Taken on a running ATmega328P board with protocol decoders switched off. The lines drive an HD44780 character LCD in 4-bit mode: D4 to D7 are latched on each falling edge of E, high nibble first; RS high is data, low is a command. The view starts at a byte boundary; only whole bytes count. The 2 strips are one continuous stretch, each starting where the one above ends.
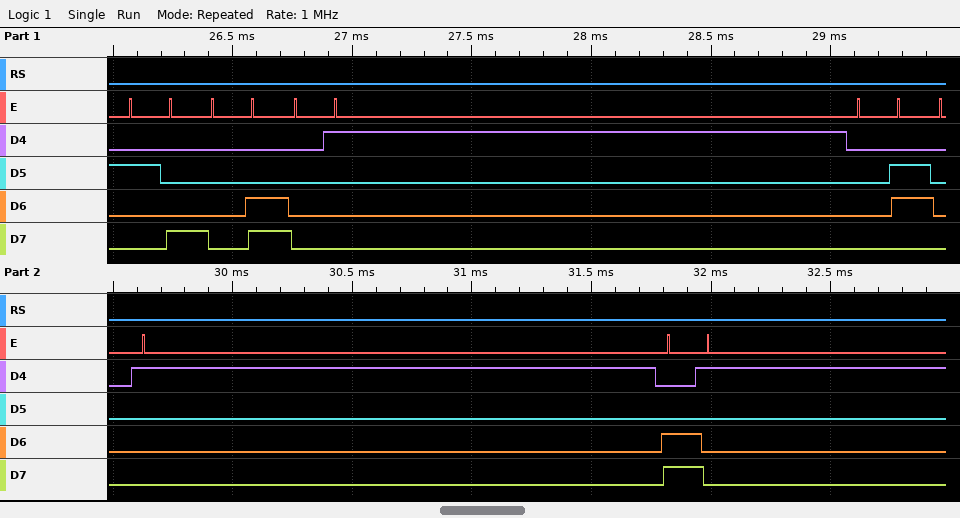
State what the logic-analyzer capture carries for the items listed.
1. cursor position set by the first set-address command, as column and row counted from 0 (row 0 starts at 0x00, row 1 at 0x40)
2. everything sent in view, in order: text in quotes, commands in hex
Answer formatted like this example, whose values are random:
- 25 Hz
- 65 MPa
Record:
- column 1, row 1
- 0x28 0x0C 0x01 0x06 0x01 0xC1
